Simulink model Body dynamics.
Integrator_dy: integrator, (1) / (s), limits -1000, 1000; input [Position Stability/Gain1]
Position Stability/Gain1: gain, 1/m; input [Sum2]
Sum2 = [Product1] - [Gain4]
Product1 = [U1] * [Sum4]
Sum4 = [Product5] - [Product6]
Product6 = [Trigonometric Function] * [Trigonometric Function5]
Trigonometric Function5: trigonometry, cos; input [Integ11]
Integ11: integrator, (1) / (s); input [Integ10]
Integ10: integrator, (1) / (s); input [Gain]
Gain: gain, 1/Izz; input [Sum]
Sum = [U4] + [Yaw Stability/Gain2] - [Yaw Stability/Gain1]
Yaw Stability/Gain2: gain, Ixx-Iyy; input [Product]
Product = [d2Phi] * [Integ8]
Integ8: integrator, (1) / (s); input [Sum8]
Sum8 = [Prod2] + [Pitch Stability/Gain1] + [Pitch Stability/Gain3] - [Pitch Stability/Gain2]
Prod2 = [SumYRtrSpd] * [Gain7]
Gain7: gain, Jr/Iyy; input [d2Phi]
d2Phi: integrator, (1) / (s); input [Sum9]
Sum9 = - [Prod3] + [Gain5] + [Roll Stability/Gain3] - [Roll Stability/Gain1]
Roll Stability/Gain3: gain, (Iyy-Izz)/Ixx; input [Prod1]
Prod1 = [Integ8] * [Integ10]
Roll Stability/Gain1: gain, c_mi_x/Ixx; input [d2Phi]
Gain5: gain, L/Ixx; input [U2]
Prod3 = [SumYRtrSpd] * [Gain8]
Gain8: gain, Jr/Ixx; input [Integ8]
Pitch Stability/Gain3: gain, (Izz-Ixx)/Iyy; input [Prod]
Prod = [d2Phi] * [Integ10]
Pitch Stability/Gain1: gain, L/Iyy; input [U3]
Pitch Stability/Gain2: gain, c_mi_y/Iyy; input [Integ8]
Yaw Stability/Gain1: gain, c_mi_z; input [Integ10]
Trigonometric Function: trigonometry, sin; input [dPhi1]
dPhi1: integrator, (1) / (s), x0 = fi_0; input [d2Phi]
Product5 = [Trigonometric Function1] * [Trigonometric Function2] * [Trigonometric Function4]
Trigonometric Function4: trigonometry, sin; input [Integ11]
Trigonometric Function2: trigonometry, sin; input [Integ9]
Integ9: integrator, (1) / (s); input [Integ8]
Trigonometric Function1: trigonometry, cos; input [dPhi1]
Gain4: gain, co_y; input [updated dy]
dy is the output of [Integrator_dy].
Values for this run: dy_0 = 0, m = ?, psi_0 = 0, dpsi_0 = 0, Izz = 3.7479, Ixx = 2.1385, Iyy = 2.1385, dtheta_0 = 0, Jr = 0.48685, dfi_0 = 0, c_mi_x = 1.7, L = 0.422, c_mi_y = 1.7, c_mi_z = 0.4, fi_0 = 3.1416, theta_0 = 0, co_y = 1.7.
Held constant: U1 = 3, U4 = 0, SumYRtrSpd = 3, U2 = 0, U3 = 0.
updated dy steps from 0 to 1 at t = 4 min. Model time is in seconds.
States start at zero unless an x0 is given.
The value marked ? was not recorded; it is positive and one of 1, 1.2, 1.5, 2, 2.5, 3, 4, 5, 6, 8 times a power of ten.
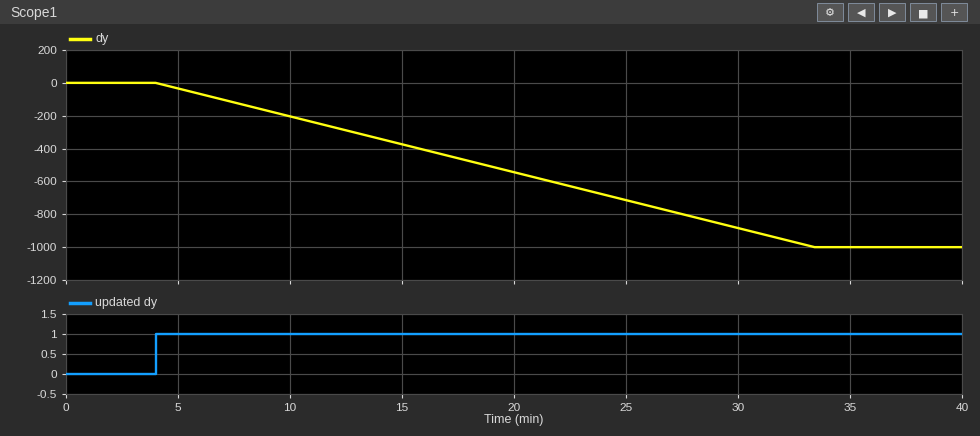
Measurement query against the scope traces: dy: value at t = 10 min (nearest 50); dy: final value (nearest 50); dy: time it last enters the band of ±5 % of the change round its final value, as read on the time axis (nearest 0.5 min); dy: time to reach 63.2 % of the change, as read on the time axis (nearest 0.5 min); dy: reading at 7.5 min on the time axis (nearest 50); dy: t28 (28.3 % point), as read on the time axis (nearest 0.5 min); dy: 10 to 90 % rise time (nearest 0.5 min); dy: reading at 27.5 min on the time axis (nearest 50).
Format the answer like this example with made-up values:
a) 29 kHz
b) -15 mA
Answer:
a) -200
b) -1000
c) 32.0 min
d) 22.5 min
e) -100
f) 12.5 min
g) 23.5 min
h) -800
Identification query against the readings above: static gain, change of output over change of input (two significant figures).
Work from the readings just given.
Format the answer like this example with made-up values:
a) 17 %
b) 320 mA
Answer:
a) -1000
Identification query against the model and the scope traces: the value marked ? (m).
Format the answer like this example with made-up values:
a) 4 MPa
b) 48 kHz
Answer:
a) 3
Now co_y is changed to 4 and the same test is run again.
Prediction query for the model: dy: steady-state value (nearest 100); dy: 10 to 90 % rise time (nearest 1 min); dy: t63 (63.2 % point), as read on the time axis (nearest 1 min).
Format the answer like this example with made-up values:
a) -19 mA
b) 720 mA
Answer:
a) -1000
b) 10 min
c) 12 min
